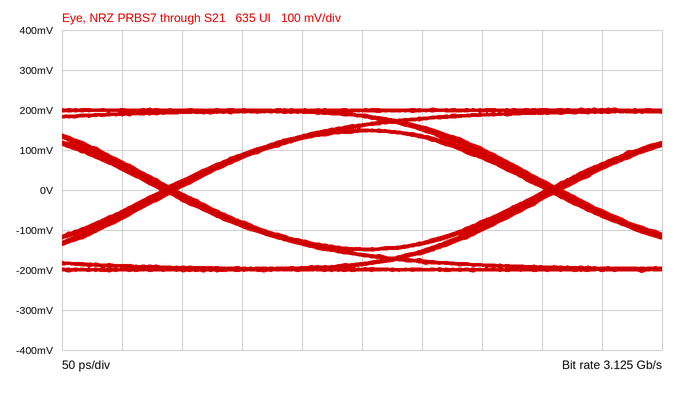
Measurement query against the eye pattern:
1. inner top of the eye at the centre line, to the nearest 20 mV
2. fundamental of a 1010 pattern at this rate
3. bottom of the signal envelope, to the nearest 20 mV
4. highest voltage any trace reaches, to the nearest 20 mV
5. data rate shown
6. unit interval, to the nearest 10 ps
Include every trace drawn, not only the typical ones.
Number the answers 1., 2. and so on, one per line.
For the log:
1. 140 mV
2. 1.5625 GHz
3. -200 mV
4. 200 mV
5. 3.125 Gb/s
6. 320 ps
